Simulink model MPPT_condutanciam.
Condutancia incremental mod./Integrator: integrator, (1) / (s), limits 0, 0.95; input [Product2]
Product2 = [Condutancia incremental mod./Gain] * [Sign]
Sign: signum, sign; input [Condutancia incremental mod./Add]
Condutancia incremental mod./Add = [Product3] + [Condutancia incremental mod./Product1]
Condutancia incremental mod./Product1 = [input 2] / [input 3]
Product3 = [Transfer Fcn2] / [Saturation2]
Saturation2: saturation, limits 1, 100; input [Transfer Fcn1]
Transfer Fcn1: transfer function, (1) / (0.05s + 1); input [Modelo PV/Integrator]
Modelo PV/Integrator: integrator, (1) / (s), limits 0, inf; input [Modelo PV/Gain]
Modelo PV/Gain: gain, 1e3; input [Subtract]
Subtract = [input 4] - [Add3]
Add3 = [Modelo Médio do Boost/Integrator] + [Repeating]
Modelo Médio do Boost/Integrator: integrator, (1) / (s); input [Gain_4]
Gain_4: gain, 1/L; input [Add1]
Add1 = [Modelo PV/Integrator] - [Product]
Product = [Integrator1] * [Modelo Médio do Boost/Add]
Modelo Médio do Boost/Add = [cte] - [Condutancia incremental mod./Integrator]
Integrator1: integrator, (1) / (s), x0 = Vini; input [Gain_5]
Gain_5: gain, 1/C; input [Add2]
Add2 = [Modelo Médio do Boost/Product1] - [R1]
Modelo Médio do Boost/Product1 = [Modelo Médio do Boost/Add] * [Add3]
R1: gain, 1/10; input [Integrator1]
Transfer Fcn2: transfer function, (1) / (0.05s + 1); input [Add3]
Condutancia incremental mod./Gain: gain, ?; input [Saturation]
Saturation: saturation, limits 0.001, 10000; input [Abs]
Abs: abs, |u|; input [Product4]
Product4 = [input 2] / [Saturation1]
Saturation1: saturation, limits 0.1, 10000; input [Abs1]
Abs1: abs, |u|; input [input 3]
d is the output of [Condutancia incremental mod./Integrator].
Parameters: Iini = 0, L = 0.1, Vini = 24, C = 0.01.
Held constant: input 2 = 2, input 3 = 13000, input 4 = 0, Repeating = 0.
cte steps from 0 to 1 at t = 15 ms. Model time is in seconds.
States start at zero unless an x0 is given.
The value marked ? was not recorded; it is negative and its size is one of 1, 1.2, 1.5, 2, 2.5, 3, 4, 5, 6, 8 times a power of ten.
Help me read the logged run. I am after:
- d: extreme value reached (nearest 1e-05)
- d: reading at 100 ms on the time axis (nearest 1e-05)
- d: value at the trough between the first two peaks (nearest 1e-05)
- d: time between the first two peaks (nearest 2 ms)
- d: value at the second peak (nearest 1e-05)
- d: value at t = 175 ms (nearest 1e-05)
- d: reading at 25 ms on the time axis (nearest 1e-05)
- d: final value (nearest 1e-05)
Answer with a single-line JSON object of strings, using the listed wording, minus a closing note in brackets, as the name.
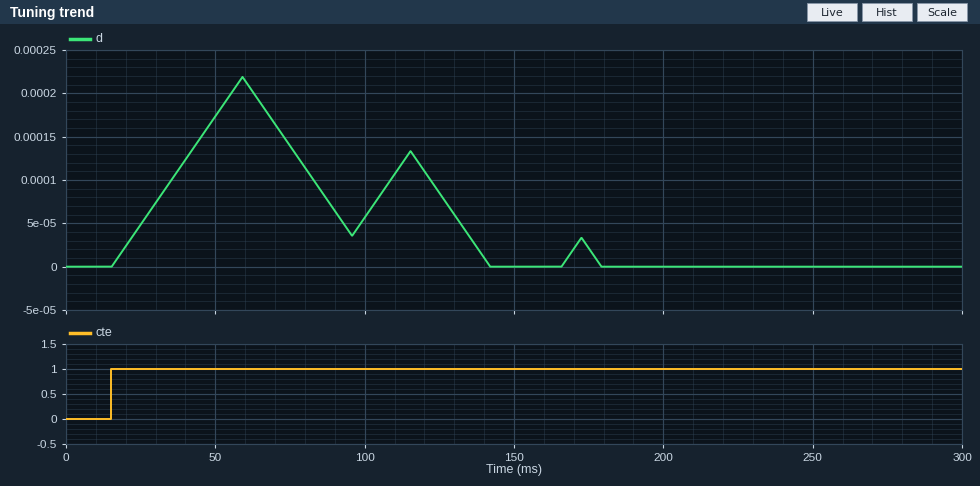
{"d: extreme value reached": "0.00022", "d: reading at 100 ms on the time axis": "0.00006", "d: value at the trough between the first two peaks": "0.00004", "d: time between the first two peaks": "56 ms", "d: value at the second peak": "0.00013", "d: value at t = 175 ms": "0.00002", "d: reading at 25 ms on the time axis": "0.00005", "d: final value": "0.00000"}
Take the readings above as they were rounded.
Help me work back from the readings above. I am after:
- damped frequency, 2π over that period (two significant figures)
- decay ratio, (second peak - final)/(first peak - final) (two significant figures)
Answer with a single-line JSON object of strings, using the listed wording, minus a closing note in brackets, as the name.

{"damped frequency, 2π over that period": "0.11 rad/ms", "decay ratio, (second peak - final)/(first peak - final)": "0.59"}
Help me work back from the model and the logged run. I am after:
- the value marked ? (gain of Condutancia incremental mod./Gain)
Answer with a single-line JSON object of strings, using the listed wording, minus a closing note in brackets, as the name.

{"the value marked ?": "-5"}
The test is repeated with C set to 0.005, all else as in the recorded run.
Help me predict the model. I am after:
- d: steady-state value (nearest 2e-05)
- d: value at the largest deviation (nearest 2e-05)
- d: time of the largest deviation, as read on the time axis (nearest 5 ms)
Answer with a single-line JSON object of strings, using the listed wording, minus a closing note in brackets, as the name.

{"d: steady-state value": "0.00000", "d: value at the largest deviation": "0.00020", "d: time of the largest deviation, as read on the time axis": "55 ms"}
